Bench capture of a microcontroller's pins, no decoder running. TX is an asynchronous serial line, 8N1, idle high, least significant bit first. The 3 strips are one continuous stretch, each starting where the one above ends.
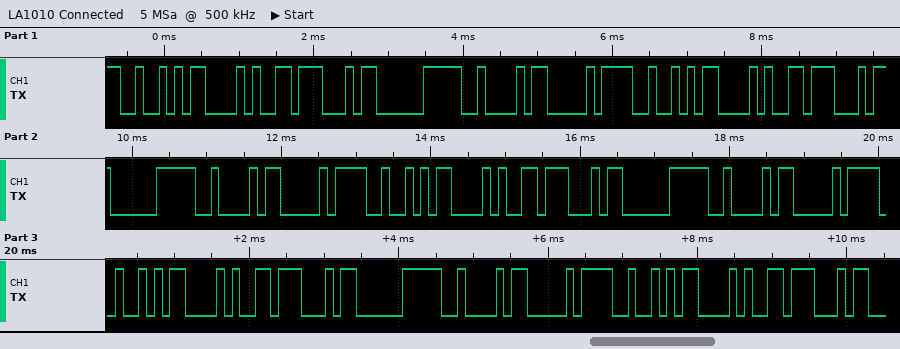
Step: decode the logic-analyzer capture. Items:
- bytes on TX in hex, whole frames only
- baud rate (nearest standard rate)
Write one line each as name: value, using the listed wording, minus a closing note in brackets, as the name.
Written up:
bytes on TX in hex, whole frames only: 0x52 0x28 0x47 0xE0 0x42 0xD0 0x52 0x28 0x47 0xE0 0x42 0xD0 0x52 0x28 0x47 0xE0 0x42 0xD0 0x52 0x28 0x47 0xE0 0x42 0xD0 0x52 0x28 0x47
baud rate: 9600 baud
